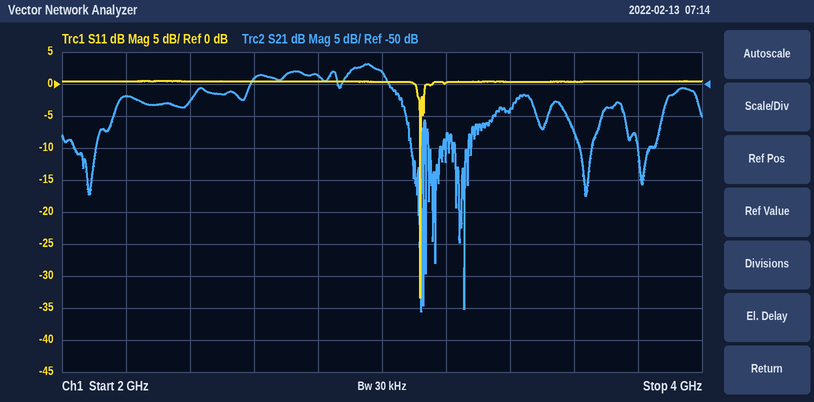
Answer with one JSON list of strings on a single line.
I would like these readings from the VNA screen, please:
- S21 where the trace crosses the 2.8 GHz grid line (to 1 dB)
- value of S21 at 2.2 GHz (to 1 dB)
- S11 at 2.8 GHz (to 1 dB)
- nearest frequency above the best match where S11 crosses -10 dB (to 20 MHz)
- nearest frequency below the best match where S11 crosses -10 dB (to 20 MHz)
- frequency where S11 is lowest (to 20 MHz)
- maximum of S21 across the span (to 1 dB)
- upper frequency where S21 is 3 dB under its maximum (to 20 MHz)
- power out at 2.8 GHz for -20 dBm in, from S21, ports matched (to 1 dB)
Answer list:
["-49 dB", "-52 dB", "0 dB", "3.12 GHz", "3.12 GHz", "3.12 GHz", "-47 dB", "3.02 GHz", "-69 dBm"]
